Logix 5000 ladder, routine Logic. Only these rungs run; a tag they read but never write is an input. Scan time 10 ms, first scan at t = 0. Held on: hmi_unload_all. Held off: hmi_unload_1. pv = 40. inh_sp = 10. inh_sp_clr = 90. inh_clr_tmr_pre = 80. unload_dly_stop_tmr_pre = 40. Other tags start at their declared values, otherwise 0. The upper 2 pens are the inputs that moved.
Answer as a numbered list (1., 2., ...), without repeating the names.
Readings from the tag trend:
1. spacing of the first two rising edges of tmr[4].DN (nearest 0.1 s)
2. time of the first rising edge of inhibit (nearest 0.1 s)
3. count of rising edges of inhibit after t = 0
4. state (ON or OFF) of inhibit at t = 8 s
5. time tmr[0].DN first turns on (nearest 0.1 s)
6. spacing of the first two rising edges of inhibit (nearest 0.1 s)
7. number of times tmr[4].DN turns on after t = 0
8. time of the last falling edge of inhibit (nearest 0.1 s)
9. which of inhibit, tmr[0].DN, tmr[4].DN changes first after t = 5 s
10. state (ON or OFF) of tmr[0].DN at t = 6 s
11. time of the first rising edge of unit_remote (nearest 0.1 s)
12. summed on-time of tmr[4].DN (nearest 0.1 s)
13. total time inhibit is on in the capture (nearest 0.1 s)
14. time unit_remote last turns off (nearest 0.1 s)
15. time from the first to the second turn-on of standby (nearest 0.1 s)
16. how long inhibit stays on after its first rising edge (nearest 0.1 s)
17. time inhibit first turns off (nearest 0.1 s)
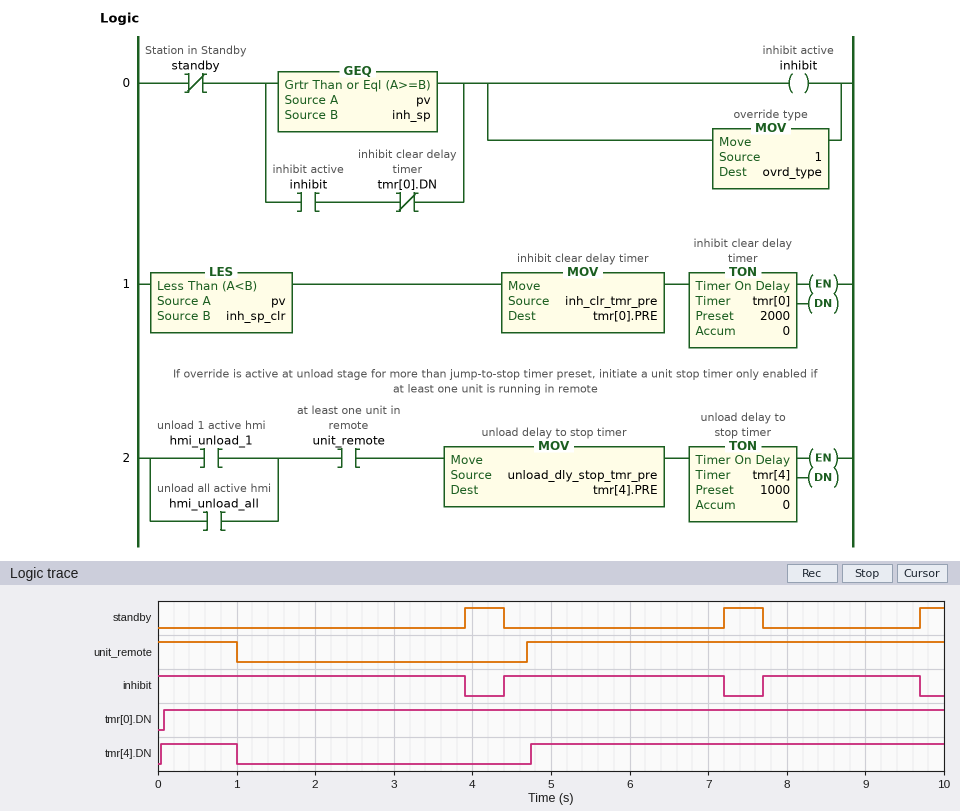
1. 4.7 s
2. 4.4 s
3. 2
4. ON
5. 0.1 s
6. 3.3 s
7. 2
8. 9.7 s
9. inhibit
10. ON
11. 4.7 s
12. 6.2 s
13. 8.7 s
14. 1.0 s
15. 3.3 s
16. 2.8 s
17. 3.9 s
